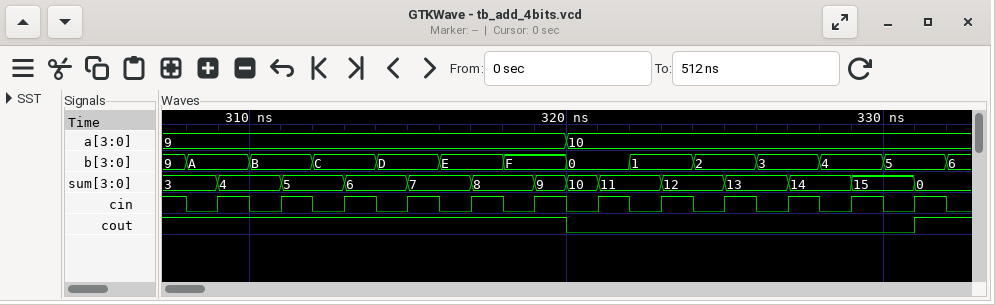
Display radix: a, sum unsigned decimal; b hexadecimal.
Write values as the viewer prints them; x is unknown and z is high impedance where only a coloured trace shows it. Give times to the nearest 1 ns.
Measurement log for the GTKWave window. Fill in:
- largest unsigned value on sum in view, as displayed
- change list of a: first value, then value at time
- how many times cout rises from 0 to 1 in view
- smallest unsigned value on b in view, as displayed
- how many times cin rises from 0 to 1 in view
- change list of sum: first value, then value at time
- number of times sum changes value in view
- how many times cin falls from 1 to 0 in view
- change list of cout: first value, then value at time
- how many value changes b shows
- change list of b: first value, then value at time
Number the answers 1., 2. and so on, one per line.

1. 15
2. 9, 10 at 320 ns
3. 1
4. 0
5. 12
6. 3, 4 at 309 ns, 5 at 311 ns, 6 at 313 ns, 7 at 315 ns, 8 at 317 ns, 9 at 319 ns, 10 at 320 ns, 11 at 321 ns, 12 at 323 ns, 13 at 325 ns, 14 at 327 ns, 15 at 329 ns, 0 at 331 ns
7. 13
8. 13
9. 1, 0 at 320 ns, 1 at 331 ns
10. 13
11. 9, A at 308 ns, B at 310 ns, C at 312 ns, D at 314 ns, E at 316 ns, F at 318 ns, 0 at 320 ns, 1 at 322 ns, 2 at 324 ns, 3 at 326 ns, 4 at 328 ns, 5 at 330 ns, 6 at 332 ns
